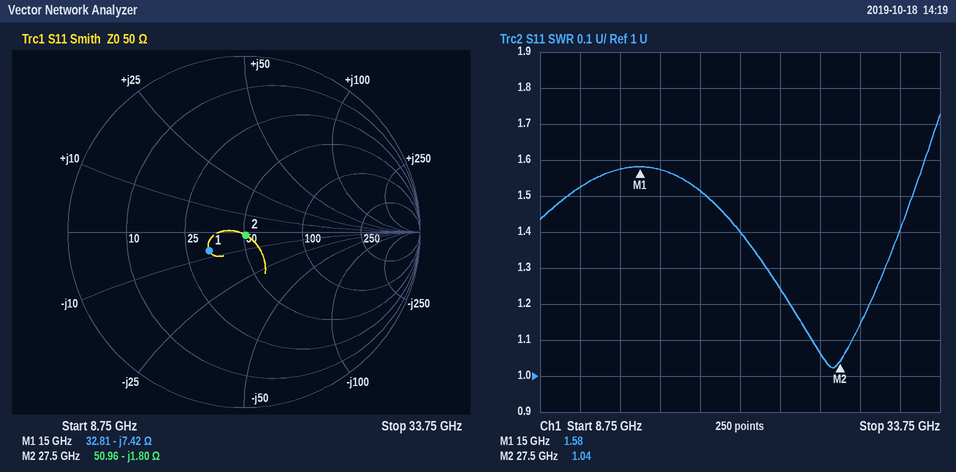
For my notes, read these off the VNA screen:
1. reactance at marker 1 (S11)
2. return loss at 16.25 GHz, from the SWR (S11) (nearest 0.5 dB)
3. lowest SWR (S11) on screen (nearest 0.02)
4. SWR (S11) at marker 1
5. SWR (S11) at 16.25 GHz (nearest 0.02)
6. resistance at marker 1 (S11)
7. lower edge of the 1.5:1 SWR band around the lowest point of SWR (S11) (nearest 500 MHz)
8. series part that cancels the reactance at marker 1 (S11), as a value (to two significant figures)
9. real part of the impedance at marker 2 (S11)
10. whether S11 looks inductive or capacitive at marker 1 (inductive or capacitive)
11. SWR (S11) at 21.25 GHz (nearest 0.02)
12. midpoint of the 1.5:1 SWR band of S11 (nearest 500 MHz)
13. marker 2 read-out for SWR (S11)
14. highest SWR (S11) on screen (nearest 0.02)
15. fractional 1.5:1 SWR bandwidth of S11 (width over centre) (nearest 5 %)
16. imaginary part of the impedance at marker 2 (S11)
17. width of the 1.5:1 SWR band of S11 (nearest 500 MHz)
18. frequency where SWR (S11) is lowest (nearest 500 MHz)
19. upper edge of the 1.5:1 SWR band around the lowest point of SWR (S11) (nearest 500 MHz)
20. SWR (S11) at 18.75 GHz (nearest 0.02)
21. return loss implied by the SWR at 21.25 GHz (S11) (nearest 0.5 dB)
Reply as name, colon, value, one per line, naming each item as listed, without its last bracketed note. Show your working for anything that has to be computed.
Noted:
reactance at marker 1: -7.42 Ω
return loss at 16.25 GHz, from the SWR (S11): −20 log10((1.58 − 1)/(1.58 + 1)) ≈ 13.0 dB
lowest SWR (S11) on screen: 1.02
SWR (S11) at marker 1: 1.58
SWR (S11) at 16.25 GHz: 1.58
resistance at marker 1: 32.81 Ω
lower edge of the 1.5:1 SWR band around the lowest point of SWR (S11): 19.0 GHz
series part that cancels the reactance at marker 1 (S11), as a value: L = 7.42 Ω/(2π × 15 GHz) ≈ 79 pH
real part of the impedance at marker 2: 50.96 Ω
whether S11 looks inductive or capacitive at marker 1: capacitive
SWR (S11) at 21.25 GHz: 1.40
midpoint of the 1.5:1 SWR band of S11: 25.5 GHz
marker 2 read-out for SWR: 1.04
highest SWR (S11) on screen: 1.72
fractional 1.5:1 SWR bandwidth of S11 (width over centre): 13 GHz / 25.5 GHz ≈ 51.0 %, so 50 % to the nearest 5 %
imaginary part of the impedance at marker 2: -1.80 Ω
width of the 1.5:1 SWR band of S11: 32.0 GHz − 19.0 GHz = 13.0 GHz
frequency where SWR (S11) is lowest: 27.0 GHz
upper edge of the 1.5:1 SWR band around the lowest point of SWR (S11): 32.0 GHz
SWR (S11) at 18.75 GHz: 1.52
return loss implied by the SWR at 21.25 GHz (S11): −20 log10((1.4 − 1)/(1.4 + 1)) ≈ 15.6 dB, so 15.5 dB to the nearest 0.5 dB
